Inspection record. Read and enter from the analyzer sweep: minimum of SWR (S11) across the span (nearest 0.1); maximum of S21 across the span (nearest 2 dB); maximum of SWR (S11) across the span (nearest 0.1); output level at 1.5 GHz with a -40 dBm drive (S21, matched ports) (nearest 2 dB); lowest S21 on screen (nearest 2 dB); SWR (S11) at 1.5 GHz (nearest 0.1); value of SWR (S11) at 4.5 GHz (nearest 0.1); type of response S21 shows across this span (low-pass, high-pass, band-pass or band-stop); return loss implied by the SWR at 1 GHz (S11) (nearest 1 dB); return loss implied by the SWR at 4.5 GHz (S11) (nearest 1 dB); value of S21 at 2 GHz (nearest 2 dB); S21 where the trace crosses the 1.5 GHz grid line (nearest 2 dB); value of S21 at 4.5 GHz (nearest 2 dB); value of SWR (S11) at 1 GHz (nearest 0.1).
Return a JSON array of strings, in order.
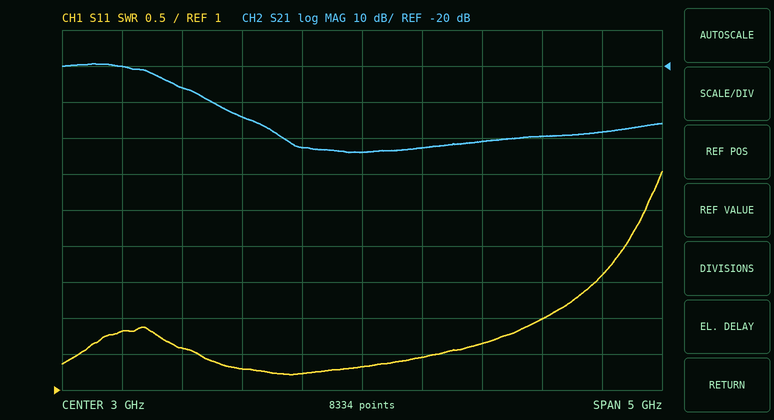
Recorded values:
["1.2", "-20 dB", "4.0", "-66 dBm", "-44 dB", "1.6", "2.0", "low-pass", "11 dB", "10 dB", "-34 dB", "-26 dB", "-40 dB", "1.8"]
